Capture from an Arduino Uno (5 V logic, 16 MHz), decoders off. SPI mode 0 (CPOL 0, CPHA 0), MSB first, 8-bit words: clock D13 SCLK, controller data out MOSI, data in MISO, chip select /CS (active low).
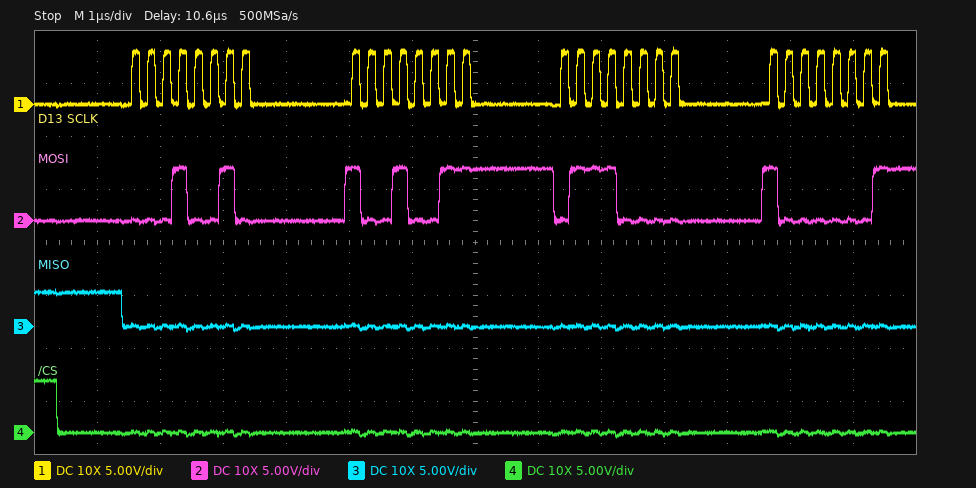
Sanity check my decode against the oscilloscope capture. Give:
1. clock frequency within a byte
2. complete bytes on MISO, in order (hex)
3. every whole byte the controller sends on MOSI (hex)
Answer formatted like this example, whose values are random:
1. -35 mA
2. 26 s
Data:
1. 4 MHz
2. 00 00 00 00
3. 12 93 70 81
